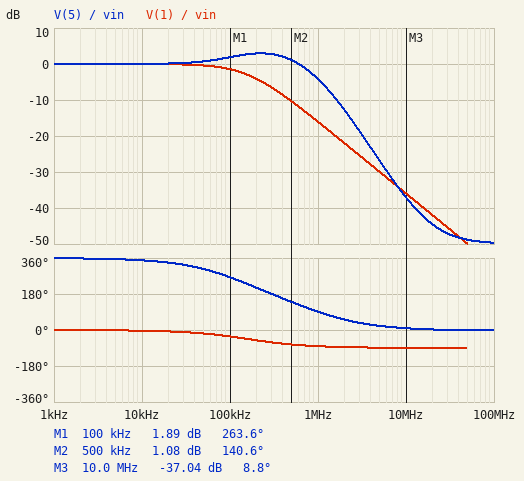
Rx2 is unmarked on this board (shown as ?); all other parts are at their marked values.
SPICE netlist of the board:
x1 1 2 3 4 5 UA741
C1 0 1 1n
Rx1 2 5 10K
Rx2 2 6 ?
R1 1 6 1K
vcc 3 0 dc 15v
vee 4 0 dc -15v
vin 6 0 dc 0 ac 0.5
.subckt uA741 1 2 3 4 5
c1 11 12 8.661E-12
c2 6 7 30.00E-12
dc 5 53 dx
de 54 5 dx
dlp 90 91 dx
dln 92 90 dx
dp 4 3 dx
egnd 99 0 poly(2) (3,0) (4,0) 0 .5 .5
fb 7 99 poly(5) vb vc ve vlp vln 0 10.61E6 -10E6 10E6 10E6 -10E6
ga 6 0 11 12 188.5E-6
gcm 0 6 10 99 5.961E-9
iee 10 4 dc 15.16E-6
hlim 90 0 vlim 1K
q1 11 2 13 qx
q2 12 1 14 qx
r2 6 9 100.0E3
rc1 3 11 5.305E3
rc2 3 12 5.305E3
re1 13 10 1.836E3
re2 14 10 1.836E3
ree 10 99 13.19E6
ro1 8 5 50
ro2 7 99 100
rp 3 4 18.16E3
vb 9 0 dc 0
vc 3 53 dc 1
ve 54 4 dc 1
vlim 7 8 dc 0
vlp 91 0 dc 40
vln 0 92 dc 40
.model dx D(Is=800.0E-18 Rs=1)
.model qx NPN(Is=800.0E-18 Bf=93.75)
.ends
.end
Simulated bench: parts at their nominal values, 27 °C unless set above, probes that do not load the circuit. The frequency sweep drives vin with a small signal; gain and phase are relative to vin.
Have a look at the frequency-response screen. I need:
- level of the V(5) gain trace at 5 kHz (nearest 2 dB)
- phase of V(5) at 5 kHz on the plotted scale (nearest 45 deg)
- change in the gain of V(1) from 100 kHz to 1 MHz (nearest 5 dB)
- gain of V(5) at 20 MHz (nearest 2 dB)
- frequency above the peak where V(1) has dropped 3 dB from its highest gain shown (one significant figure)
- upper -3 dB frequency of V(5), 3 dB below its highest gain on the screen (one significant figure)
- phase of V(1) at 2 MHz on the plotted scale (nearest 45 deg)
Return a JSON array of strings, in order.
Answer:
["0 dB", "360 deg", "-15 dB", "-44 dB", "200 kHz", "600 kHz", "-90 deg"]
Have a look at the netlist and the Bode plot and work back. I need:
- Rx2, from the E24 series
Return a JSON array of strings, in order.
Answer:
["5.6 kΩ"]
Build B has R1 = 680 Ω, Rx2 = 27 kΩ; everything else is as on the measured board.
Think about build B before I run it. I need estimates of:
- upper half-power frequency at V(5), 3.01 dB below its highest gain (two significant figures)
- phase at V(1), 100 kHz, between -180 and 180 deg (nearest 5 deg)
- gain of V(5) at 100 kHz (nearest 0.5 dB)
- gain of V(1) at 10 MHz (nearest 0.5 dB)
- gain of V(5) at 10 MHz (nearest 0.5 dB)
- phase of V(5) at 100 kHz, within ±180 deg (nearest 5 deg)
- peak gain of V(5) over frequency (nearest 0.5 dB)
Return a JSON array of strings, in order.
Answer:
["270 kHz", "-25 deg", "-0.5 dB", "-32.5 dB", "-44.5 dB", "-40 deg", "0 dB"]
